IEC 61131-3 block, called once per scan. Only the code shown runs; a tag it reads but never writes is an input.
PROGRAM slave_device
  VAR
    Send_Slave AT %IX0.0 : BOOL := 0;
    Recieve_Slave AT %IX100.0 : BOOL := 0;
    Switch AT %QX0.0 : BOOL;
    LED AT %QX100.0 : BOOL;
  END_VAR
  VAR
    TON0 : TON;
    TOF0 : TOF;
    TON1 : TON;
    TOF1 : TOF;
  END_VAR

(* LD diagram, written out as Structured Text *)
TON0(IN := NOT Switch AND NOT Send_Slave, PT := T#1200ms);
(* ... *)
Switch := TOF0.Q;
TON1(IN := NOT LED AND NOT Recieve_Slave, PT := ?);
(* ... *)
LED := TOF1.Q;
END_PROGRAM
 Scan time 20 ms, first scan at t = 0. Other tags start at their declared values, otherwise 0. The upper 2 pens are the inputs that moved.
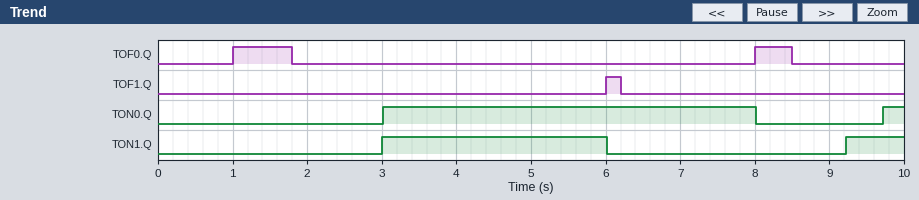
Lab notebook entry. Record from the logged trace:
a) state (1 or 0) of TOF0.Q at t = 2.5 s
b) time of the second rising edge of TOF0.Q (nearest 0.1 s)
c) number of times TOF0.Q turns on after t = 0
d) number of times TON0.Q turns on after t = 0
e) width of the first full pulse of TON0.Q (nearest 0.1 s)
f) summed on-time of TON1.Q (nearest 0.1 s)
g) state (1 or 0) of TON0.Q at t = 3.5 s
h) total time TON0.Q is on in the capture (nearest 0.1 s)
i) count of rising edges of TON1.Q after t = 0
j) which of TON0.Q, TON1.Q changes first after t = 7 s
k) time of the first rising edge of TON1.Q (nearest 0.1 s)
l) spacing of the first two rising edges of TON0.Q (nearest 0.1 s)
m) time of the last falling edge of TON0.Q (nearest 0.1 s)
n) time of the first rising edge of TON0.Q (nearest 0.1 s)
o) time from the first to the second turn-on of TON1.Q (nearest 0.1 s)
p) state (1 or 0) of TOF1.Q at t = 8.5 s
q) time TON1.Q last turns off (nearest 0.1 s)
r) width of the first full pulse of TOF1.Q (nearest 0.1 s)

0
8.0 s
2
2
5.0 s
3.8 s
1
5.3 s
2
TON0.Q
3.0 s
6.7 s
8.0 s
3.0 s
6.2 s
0
6.0 s
0.2 s
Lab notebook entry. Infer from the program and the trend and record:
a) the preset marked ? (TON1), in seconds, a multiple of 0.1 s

3.0 s
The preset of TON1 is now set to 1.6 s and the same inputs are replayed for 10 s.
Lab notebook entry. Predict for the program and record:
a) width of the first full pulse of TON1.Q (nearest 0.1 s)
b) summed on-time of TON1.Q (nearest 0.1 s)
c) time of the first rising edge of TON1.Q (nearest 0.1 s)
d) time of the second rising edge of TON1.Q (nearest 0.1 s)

4.4 s
6.6 s
1.6 s
7.8 s
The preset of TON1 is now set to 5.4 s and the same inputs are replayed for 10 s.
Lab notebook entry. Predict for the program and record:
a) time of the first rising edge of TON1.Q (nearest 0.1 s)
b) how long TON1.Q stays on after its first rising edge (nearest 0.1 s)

5.4 s
0.6 s
